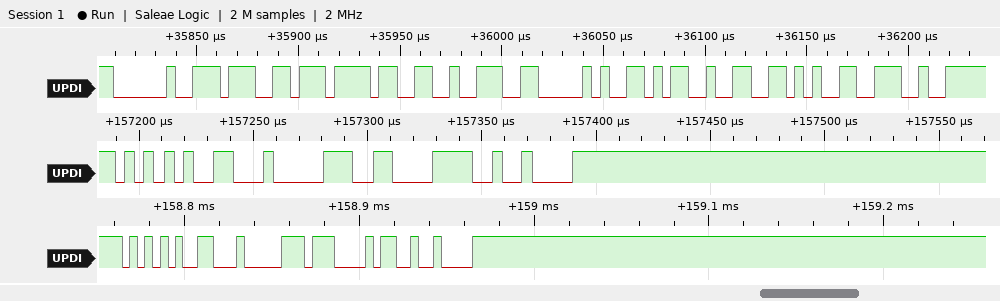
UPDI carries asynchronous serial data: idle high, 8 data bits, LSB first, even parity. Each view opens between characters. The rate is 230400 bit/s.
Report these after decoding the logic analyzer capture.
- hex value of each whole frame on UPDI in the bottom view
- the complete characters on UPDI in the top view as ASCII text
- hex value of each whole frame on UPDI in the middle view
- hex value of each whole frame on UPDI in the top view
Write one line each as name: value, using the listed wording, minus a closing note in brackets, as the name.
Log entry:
hex value of each whole frame on UPDI in the bottom view: 55, 04, 87, 12
the complete characters on UPDI in the top view as ASCII text: " gorPMVN"
hex value of each whole frame on UPDI in the middle view: 55, 04, 86, 12
hex value of each whole frame on UPDI in the top view: 20, 67, 6F, 72, 50, 4D, 56, 4E
